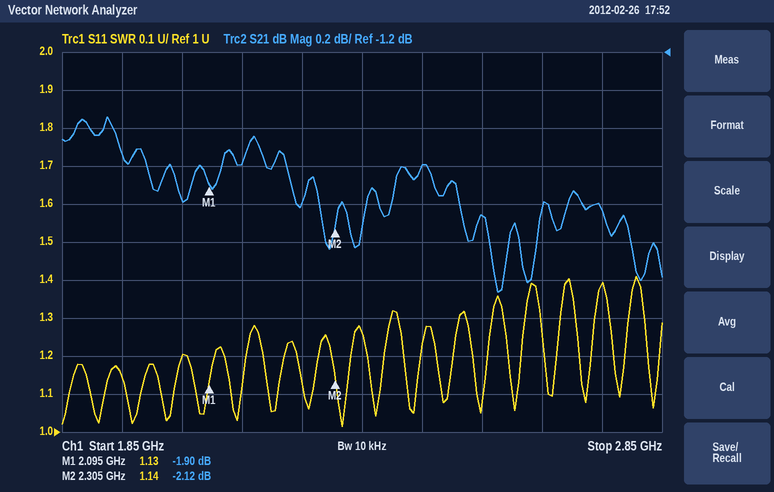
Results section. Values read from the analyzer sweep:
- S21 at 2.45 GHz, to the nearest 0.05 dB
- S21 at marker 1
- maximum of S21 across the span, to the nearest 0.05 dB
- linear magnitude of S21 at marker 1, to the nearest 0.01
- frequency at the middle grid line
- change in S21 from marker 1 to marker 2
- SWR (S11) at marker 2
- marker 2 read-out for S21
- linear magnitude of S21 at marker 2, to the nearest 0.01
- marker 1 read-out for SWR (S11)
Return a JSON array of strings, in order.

["-1.80 dB", "-1.90 dB", "-1.55 dB", "0.80", "2.35 GHz", "-0.22 dB", "1.14", "-2.12 dB", "0.78", "1.13"]
